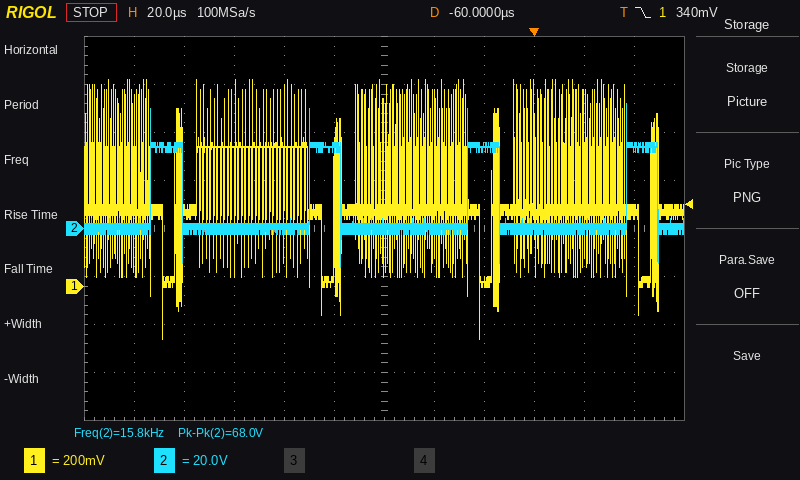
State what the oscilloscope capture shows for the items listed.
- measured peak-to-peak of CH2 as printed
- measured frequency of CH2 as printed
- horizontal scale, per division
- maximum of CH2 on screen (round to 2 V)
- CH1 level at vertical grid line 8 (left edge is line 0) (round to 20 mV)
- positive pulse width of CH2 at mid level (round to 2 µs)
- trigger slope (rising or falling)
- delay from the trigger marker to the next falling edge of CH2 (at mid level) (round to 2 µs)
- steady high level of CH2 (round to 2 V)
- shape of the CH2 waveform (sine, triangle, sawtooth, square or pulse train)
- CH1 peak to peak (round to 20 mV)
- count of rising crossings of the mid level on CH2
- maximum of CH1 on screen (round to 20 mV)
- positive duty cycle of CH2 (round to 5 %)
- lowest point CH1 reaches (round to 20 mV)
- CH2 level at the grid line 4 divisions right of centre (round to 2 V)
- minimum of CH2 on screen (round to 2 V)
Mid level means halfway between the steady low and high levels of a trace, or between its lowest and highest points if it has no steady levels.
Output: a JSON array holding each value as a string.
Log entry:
["68.0 V", "15.8 kHz", "20 µs", "52 V", "20 mV", "12 µs", "falling", "50 µs", "34 V", "pulse train", "1.08 V", "4", "860 mV", "20 %", "-220 mV", "0 V", "-16 V"]
